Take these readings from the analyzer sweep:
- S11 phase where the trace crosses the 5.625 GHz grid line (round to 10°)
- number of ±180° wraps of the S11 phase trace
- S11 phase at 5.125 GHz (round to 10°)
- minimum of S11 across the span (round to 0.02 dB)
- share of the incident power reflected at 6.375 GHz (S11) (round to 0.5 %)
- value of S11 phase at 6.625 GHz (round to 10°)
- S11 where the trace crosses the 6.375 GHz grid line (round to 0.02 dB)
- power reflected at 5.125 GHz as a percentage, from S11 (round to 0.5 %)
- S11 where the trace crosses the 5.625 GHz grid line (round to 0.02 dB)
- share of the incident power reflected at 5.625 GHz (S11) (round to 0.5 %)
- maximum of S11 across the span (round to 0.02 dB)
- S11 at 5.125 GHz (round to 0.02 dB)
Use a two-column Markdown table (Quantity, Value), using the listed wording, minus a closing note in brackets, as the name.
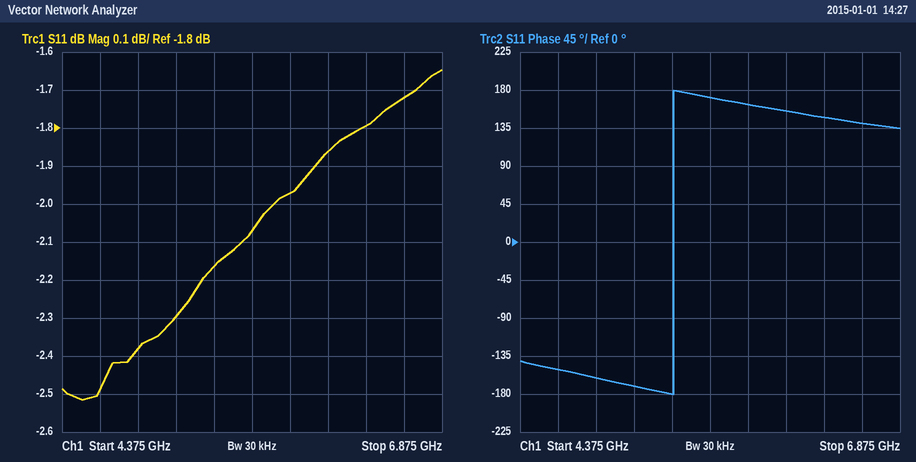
| Quantity | Value |
|---|---|
| S11 phase where the trace crosses the 5.625 GHz grid line | 170° |
| number of ±180° wraps of the S11 phase trace | 1 |
| S11 phase at 5.125 GHz | -170° |
| minimum of S11 across the span | -2.52 dB |
| share of the incident power reflected at 6.375 GHz (S11) | 66.0 % |
| value of S11 phase at 6.625 GHz | 140° |
| S11 where the trace crosses the 6.375 GHz grid line | -1.80 dB |
| power reflected at 5.125 GHz as a percentage, from S11 | 59.0 % |
| S11 where the trace crosses the 5.625 GHz grid line | -2.08 dB |
| share of the incident power reflected at 5.625 GHz (S11) | 62.0 % |
| maximum of S11 across the span | -1.64 dB |
| S11 at 5.125 GHz | -2.30 dB |
